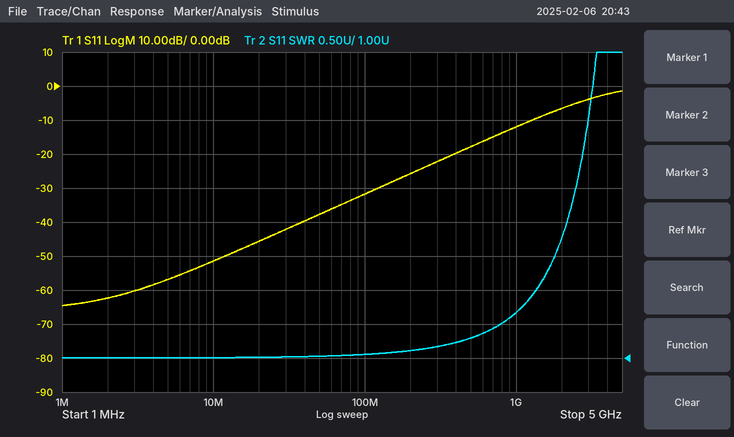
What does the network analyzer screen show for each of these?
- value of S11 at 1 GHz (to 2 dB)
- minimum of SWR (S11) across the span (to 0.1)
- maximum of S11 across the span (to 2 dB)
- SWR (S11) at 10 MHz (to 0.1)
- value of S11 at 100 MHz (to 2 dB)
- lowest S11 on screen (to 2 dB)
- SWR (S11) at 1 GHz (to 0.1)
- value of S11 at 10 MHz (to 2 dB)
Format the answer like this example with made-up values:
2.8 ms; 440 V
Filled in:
-12 dB; 1.0; -2 dB; 1.0; -32 dB; -64 dB; 1.7; -52 dB
